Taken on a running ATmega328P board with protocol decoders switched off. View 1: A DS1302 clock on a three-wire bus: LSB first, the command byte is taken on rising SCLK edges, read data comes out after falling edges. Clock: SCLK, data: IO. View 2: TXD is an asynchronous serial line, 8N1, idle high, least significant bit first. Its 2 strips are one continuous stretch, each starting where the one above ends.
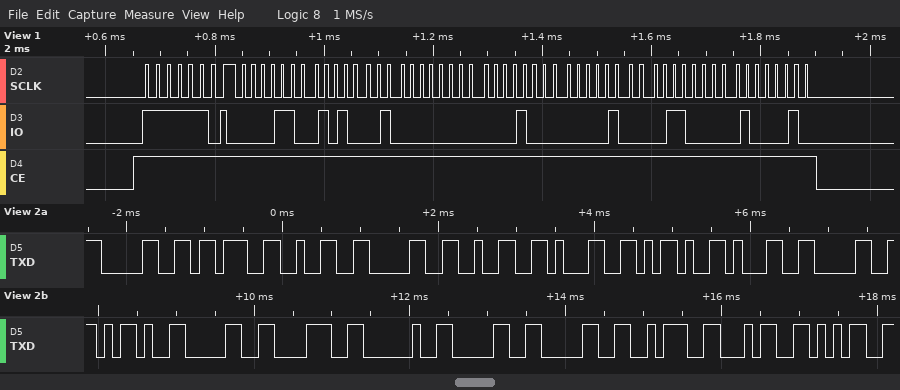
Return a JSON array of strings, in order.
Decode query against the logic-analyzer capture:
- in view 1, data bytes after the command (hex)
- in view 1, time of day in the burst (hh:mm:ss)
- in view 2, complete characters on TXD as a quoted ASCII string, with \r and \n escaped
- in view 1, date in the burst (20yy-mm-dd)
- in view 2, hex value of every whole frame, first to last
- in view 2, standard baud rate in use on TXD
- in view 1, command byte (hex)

["30 45 00 08 10 06 21", "00:45:30", "\"0;2021-10-08 00:45\"", "2021-10-08", "30 3B 32 30 32 31 2D 31 30 2D 30 38 20 30 30 3A 34 35", "9600 baud", "0xBF"]
